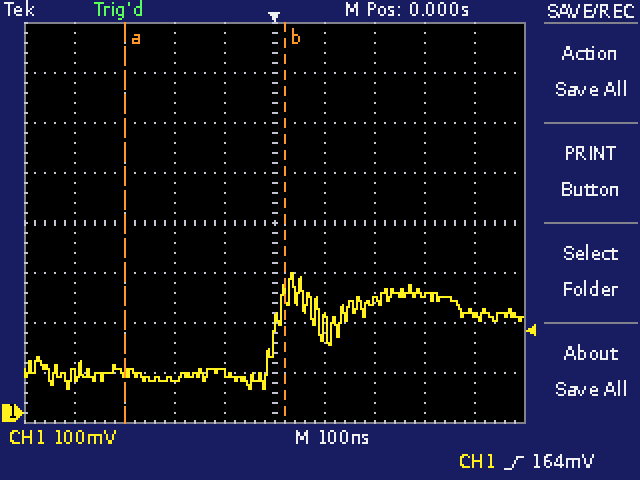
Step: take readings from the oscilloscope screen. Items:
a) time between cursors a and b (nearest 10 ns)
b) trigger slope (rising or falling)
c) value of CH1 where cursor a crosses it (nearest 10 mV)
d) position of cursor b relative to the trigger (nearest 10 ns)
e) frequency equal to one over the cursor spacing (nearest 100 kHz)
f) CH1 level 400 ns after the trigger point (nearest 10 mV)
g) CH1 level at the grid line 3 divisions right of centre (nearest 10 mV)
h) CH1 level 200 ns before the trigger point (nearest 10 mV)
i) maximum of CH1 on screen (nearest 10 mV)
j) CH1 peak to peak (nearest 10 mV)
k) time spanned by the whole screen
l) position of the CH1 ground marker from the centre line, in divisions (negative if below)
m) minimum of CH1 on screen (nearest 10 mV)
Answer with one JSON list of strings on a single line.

["320 ns", "rising", "80 mV", "+20 ns", "3.1 MHz", "200 mV", "240 mV", "70 mV", "280 mV", "230 mV", "1 µs", "-3.8 div", "50 mV"]
